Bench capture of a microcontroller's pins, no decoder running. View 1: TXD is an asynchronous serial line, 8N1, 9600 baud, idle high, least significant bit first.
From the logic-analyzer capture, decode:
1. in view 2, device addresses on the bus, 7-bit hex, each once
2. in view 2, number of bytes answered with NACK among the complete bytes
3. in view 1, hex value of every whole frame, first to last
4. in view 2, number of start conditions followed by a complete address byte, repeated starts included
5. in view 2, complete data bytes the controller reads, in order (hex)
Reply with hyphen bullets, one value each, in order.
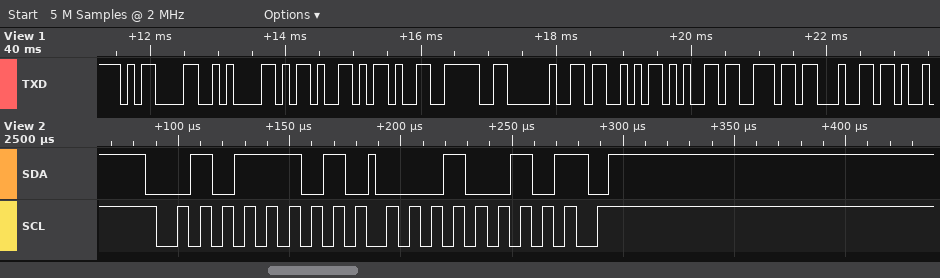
- 0x2E
- 1
- 0D 0A 2D 2D 3E 20 53 65 6E 64
- 1
- 12
